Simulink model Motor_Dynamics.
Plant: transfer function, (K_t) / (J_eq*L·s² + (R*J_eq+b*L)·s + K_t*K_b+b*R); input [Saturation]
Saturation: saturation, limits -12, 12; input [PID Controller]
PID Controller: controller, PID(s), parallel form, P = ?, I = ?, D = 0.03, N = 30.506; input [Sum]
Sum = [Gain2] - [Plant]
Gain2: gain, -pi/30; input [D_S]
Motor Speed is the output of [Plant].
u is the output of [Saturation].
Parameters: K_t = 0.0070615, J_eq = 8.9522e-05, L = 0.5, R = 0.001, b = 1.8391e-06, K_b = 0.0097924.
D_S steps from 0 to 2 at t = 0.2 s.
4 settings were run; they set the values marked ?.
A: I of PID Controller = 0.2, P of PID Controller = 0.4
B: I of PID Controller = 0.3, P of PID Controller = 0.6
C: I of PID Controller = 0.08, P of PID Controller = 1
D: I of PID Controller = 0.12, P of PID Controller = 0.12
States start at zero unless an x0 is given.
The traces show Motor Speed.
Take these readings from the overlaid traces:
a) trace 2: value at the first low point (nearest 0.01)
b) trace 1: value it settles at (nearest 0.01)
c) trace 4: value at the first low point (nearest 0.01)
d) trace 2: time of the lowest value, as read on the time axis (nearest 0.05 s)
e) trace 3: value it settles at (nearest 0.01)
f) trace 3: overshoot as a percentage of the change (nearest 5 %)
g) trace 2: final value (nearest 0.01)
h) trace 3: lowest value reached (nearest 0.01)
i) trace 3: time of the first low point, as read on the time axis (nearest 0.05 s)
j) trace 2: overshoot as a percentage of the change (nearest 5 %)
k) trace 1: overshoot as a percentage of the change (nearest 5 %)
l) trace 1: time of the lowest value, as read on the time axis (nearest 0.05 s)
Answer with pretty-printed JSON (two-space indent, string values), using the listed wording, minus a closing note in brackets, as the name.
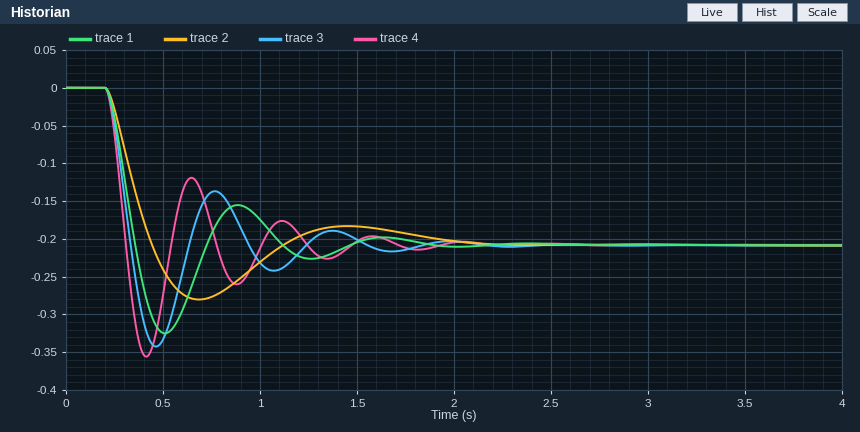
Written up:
{
  "trace 2: value at the first low point": "-0.28",
  "trace 1: value it settles at": "-0.21",
  "trace 4: value at the first low point": "-0.36",
  "trace 2: time of the lowest value, as read on the time axis": "0.70 s",
  "trace 3: value it settles at": "-0.21",
  "trace 3: overshoot as a percentage of the change": "65 %",
  "trace 2: final value": "-0.21",
  "trace 3: lowest value reached": "-0.34",
  "trace 3: time of the first low point, as read on the time axis": "0.45 s",
  "trace 2: overshoot as a percentage of the change": "35 %",
  "trace 1: overshoot as a percentage of the change": "55 %",
  "trace 1: time of the lowest value, as read on the time axis": "0.50 s"
}
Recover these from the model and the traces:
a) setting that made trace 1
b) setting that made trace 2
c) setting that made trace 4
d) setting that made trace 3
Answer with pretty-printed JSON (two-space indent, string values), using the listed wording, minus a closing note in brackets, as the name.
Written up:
{
  "setting that made trace 1": "A",
  "setting that made trace 2": "D",
  "setting that made trace 4": "C",
  "setting that made trace 3": "B"
}
